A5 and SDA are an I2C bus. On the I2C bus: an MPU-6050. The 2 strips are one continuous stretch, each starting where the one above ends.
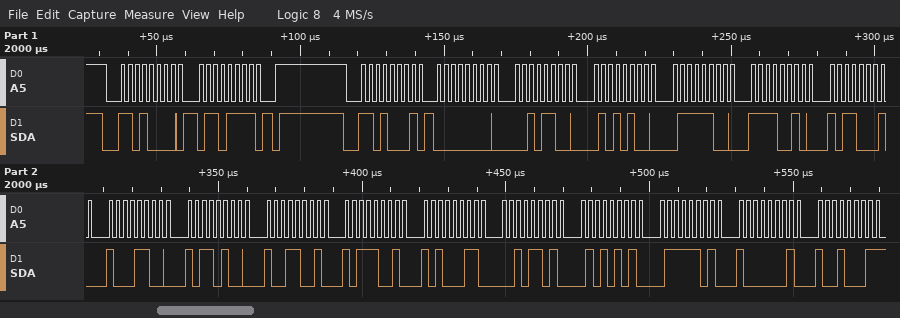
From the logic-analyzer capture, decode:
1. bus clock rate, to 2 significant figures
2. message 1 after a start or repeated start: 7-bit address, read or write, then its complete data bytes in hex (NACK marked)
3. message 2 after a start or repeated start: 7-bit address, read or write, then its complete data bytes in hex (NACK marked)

400 kHz
0x68 write: 6F
0x68 read: 00 2C 54 7C F2 B1 8C B4 99 B9 A3 2D 55 7D 81 91 NACK
